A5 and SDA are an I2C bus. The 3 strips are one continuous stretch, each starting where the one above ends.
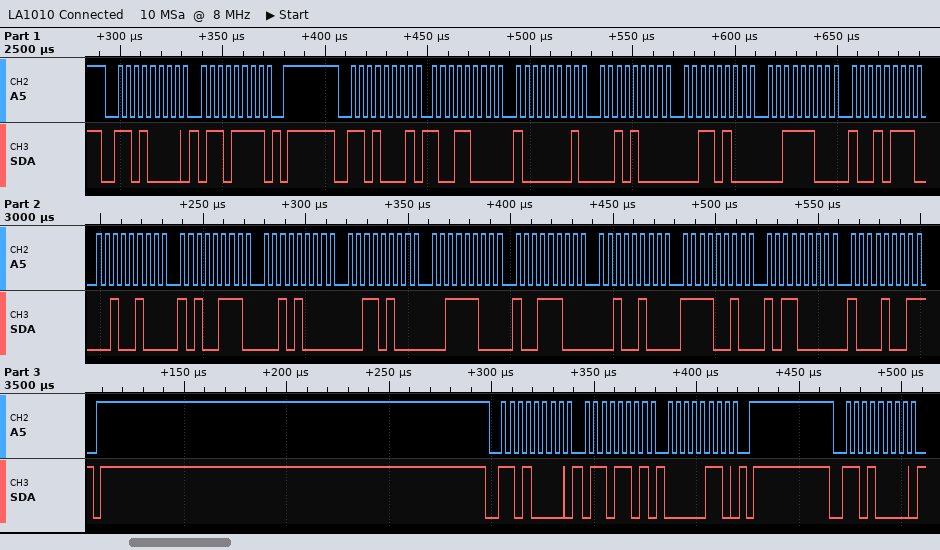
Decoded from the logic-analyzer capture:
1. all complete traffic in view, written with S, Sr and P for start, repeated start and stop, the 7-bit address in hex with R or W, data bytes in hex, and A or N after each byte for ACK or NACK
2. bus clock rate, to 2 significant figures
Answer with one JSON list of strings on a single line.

["S 68W A 6F A P S 68R A 98 A 81 A 28 A 34 A 3C A 97 A 24 A A7 A 28 A 34 A 3C A 9C A 24 A F2 A B0 A 89 N P S 68W A 6D A 06 A P S 68W A", "250 kHz"]
